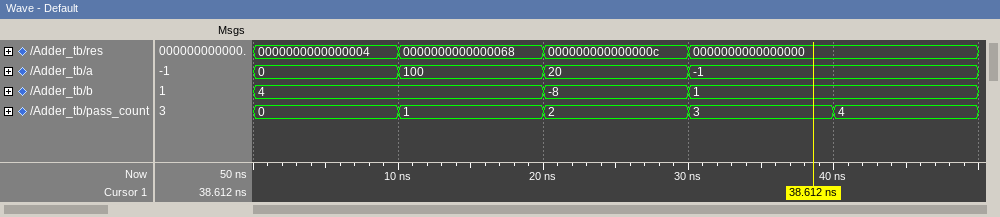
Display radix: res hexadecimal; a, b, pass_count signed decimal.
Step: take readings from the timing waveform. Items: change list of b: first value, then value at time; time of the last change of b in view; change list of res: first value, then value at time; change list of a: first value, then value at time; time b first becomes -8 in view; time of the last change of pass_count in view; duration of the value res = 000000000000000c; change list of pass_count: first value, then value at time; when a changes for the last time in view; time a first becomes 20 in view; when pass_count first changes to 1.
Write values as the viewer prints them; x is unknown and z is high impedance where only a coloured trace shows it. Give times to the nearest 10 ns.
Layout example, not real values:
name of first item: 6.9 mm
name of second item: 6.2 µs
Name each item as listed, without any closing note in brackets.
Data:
change list of b: first value, then value at time: 4, -8 at 20 ns, 1 at 30 ns
time of the last change of b in view: 30 ns
change list of res: first value, then value at time: 0000000000000004, 0000000000000068 at 10 ns, 000000000000000c at 20 ns, 0000000000000000 at 30 ns
change list of a: first value, then value at time: 0, 100 at 10 ns, 20 at 20 ns, -1 at 30 ns
time b first becomes -8 in view: 20 ns
time of the last change of pass_count in view: 40 ns
duration of the value res = 000000000000000c: 10 ns
change list of pass_count: first value, then value at time: 0, 1 at 10 ns, 2 at 20 ns, 3 at 30 ns, 4 at 40 ns
when a changes for the last time in view: 30 ns
time a first becomes 20 in view: 20 ns
when pass_count first changes to 1: 10 ns
